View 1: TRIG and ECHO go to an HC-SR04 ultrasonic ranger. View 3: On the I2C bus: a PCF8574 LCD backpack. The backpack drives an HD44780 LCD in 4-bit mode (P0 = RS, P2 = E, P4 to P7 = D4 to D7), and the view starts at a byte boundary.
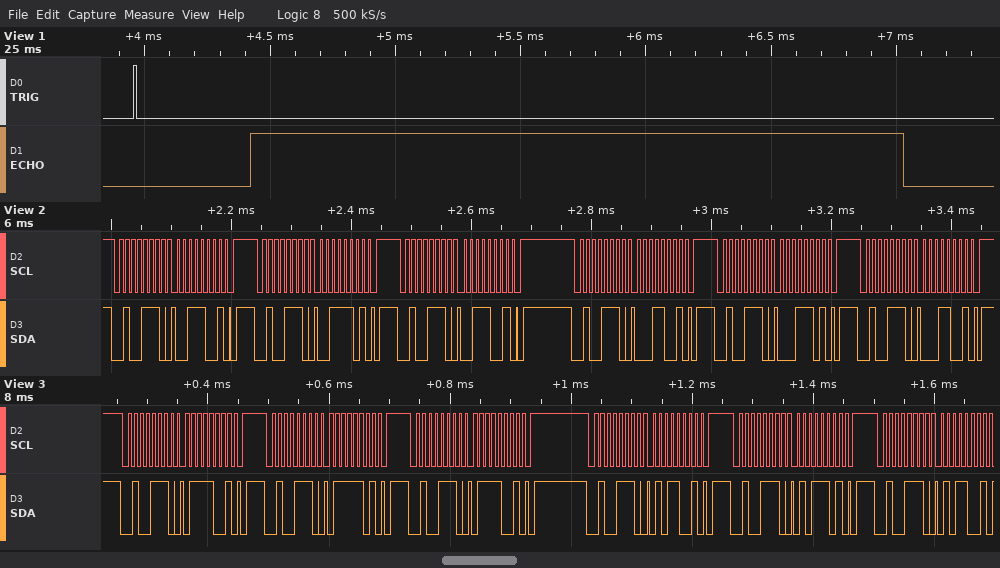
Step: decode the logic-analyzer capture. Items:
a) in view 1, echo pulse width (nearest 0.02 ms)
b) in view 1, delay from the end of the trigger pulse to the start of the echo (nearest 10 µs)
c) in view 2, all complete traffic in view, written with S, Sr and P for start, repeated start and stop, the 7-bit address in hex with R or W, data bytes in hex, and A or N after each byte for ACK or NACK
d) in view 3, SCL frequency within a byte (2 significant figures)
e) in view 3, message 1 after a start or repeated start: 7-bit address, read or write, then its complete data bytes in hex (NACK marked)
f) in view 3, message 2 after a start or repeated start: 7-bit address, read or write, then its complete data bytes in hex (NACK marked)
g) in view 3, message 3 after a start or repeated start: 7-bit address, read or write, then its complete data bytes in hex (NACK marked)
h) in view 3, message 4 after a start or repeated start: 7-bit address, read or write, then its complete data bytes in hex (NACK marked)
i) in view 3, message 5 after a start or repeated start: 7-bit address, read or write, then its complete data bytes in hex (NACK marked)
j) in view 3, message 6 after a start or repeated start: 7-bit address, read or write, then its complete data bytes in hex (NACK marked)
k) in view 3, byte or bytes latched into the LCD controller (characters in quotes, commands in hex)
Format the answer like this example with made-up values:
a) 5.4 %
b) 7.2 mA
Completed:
a) 2.60 ms
b) 460 µs
c) S 27W A 39 A P S 27W A 3D A P S 27W A 39 A P S 27W A 19 A P S 27W A 1D A P S 27W A 19 A P
d) 100 kHz
e) 0x27 write: 79
f) 0x27 write: 7D
g) 0x27 write: 79
h) 0x27 write: 59
i) 0x27 write: 5D
j) 0x27 write: 59
k) 'u'
